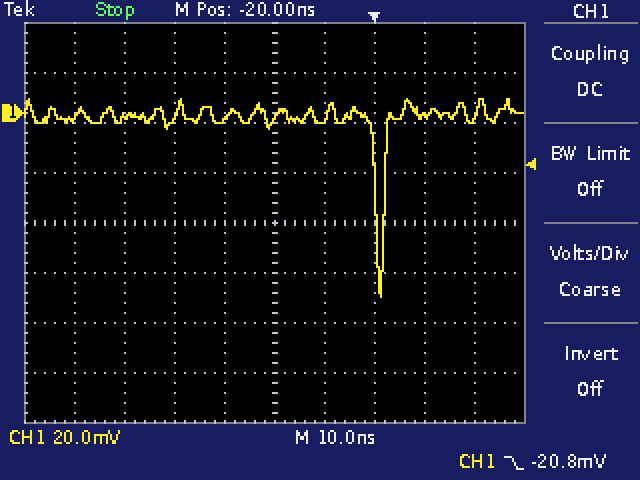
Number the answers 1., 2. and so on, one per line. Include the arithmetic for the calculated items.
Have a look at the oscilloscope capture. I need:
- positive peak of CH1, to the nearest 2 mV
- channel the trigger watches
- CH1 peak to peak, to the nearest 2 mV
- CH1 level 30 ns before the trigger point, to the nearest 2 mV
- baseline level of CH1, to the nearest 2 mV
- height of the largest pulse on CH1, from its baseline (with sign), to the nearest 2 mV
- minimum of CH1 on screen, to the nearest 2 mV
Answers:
1. 6 mV
2. CH1
3. 6 mV − (-74 mV) = 80 mV
4. -2 mV
5. -2 mV
6. -74 mV − (-2 mV) = -72 mV
7. -74 mV
